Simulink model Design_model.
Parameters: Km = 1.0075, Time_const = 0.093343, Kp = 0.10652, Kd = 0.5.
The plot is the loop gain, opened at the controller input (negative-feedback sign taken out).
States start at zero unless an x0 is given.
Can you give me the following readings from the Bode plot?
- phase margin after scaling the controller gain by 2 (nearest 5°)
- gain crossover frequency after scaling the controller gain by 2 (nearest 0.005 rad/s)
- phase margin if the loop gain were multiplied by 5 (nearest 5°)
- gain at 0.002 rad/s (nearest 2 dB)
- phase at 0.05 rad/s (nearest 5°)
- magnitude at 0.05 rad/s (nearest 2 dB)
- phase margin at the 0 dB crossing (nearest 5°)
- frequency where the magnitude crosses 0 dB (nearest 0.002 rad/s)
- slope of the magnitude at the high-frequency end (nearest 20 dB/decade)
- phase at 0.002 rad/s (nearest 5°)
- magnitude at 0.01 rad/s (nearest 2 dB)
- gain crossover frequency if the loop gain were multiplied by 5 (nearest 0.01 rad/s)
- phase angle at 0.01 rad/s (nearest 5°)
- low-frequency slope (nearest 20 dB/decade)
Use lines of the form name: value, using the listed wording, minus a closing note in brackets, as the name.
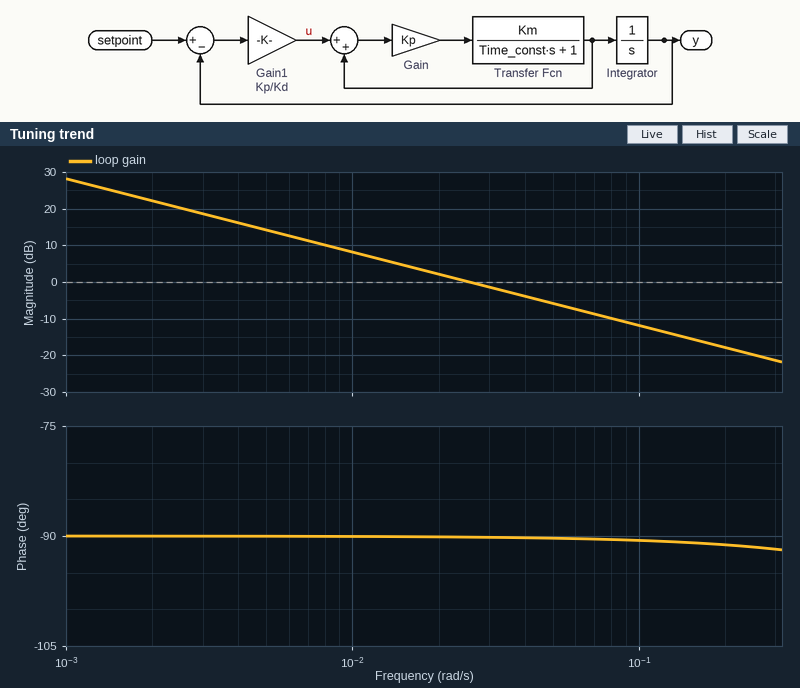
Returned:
phase margin after scaling the controller gain by 2: 90°
gain crossover frequency after scaling the controller gain by 2: 0.050 rad/s
phase margin if the loop gain were multiplied by 5: 90°
gain at 0.002 rad/s: 22 dB
phase at 0.05 rad/s: -90°
magnitude at 0.05 rad/s: -6 dB
phase margin at the 0 dB crossing: 90°
frequency where the magnitude crosses 0 dB: 0.026 rad/s
slope of the magnitude at the high-frequency end: -20 dB/decade
phase at 0.002 rad/s: -90°
magnitude at 0.01 rad/s: 8 dB
gain crossover frequency if the loop gain were multiplied by 5: 0.13 rad/s
phase angle at 0.01 rad/s: -90°
low-frequency slope: -20 dB/decade
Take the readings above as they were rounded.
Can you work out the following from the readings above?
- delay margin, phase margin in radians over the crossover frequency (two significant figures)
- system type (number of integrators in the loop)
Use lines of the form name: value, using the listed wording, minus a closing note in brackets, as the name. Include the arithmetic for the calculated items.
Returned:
delay margin, phase margin in radians over the crossover frequency: 90 × π / 180 / 0.026 = 60 s
system type: 1
